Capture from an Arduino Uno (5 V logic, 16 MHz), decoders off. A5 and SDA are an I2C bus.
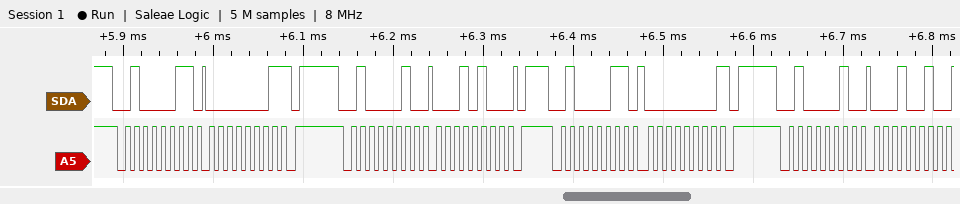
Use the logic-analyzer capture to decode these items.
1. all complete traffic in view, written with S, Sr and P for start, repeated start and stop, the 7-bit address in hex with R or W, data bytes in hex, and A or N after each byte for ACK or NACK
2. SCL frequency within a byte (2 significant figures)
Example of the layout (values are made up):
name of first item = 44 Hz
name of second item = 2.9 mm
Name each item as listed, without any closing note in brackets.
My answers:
all complete traffic in view, written with S, Sr and P for start, repeated start and stop, the 7-bit address in hex with R or W, data bytes in hex, and A or N after each byte for ACK or NACK = S 21R A 01 N P S 21W A 14 A P S 21R A 00 N P S 21W A 12 A
SCL frequency within a byte = 100 kHz
